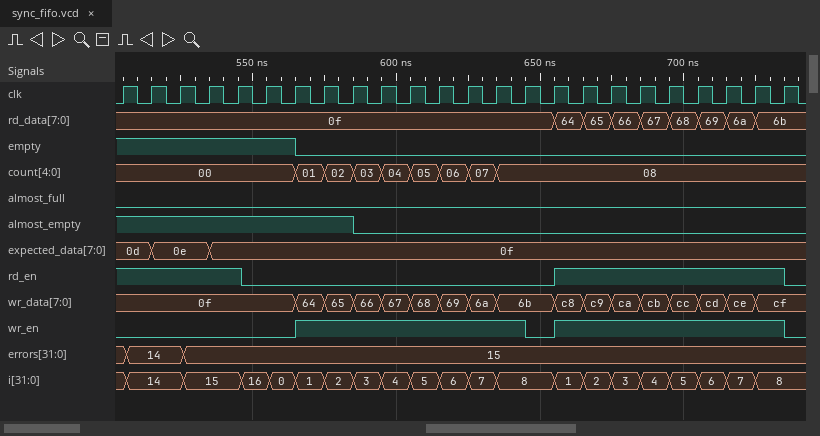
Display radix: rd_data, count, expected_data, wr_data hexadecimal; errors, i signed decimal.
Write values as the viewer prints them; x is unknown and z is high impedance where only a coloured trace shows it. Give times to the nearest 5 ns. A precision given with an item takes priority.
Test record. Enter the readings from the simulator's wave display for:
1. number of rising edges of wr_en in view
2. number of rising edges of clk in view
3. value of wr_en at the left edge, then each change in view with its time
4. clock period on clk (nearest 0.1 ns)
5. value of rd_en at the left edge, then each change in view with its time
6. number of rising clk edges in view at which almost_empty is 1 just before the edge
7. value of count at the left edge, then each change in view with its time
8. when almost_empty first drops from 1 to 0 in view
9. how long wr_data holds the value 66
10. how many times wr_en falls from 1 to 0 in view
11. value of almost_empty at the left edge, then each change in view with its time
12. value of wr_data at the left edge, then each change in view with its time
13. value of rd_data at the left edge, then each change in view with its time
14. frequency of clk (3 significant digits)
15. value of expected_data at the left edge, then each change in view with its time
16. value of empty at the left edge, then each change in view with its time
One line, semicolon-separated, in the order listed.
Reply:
2; 24; 0, 1 at 565 ns, 0 at 645 ns, 1 at 655 ns, 0 at 735 ns; 10 ns; 1, 0 at 545 ns, 1 at 655 ns, 0 at 735 ns; 9; 00, 01 at 565 ns, 02 at 575 ns, 03 at 585 ns, 04 at 595 ns, 05 at 605 ns, 06 at 615 ns, 07 at 625 ns, 08 at 635 ns; 585 ns; 10 ns; 2; 1, 0 at 585 ns; 0f, 64 at 565 ns, 65 at 575 ns, 66 at 585 ns, 67 at 595 ns, 68 at 605 ns, 69 at 615 ns, 6a at 625 ns, 6b at 635 ns, c8 at 655 ns, c9 at 665 ns, ca at 675 ns, cb at 685 ns, cc at 695 ns, cd at 705 ns, ce at 715 ns, cf at 725 ns; 0f, 64 at 655 ns, 65 at 665 ns, 66 at 675 ns, 67 at 685 ns, 68 at 695 ns, 69 at 705 ns, 6a at 715 ns, 6b at 725 ns; 100 MHz; 0d, 0e at 515 ns, 0f at 535 ns; 1, 0 at 565 ns
